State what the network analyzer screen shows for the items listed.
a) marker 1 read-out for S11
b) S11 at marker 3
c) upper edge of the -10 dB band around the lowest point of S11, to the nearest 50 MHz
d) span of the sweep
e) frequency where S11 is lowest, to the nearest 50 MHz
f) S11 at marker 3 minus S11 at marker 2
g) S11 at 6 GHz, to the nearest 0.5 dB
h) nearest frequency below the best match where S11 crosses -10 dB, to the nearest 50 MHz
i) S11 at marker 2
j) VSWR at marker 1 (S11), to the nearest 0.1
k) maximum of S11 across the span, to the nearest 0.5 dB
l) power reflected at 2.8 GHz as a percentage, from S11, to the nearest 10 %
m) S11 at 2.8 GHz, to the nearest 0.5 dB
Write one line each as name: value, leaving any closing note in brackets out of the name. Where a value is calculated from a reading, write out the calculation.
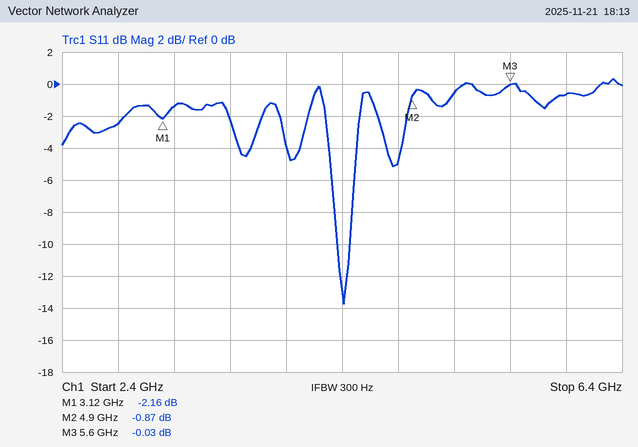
marker 1 read-out for S11: -2.16 dB
S11 at marker 3: -0.03 dB
upper edge of the -10 dB band around the lowest point of S11, to the nearest 50 MHz: 4.45 GHz
span of the sweep: 4 GHz
frequency where S11 is lowest, to the nearest 50 MHz: 4.40 GHz
S11 at marker 3 minus S11 at marker 2: -0.03 − (-0.87) = 0.84 dB
S11 at 6 GHz, to the nearest 0.5 dB: -0.5 dB
nearest frequency below the best match where S11 crosses -10 dB, to the nearest 50 MHz: 4.35 GHz
S11 at marker 2: -0.87 dB
VSWR at marker 1 (S11), to the nearest 0.1: (1 + 0.7798)/(1 − 0.7798) ≈ 8.1
maximum of S11 across the span, to the nearest 0.5 dB: 0.5 dB
power reflected at 2.8 GHz as a percentage, from S11, to the nearest 10 %: 10^(-2.5/10) ≈ 56.2 %, so 60 % to the nearest 10 %
S11 at 2.8 GHz, to the nearest 0.5 dB: -2.5 dB
